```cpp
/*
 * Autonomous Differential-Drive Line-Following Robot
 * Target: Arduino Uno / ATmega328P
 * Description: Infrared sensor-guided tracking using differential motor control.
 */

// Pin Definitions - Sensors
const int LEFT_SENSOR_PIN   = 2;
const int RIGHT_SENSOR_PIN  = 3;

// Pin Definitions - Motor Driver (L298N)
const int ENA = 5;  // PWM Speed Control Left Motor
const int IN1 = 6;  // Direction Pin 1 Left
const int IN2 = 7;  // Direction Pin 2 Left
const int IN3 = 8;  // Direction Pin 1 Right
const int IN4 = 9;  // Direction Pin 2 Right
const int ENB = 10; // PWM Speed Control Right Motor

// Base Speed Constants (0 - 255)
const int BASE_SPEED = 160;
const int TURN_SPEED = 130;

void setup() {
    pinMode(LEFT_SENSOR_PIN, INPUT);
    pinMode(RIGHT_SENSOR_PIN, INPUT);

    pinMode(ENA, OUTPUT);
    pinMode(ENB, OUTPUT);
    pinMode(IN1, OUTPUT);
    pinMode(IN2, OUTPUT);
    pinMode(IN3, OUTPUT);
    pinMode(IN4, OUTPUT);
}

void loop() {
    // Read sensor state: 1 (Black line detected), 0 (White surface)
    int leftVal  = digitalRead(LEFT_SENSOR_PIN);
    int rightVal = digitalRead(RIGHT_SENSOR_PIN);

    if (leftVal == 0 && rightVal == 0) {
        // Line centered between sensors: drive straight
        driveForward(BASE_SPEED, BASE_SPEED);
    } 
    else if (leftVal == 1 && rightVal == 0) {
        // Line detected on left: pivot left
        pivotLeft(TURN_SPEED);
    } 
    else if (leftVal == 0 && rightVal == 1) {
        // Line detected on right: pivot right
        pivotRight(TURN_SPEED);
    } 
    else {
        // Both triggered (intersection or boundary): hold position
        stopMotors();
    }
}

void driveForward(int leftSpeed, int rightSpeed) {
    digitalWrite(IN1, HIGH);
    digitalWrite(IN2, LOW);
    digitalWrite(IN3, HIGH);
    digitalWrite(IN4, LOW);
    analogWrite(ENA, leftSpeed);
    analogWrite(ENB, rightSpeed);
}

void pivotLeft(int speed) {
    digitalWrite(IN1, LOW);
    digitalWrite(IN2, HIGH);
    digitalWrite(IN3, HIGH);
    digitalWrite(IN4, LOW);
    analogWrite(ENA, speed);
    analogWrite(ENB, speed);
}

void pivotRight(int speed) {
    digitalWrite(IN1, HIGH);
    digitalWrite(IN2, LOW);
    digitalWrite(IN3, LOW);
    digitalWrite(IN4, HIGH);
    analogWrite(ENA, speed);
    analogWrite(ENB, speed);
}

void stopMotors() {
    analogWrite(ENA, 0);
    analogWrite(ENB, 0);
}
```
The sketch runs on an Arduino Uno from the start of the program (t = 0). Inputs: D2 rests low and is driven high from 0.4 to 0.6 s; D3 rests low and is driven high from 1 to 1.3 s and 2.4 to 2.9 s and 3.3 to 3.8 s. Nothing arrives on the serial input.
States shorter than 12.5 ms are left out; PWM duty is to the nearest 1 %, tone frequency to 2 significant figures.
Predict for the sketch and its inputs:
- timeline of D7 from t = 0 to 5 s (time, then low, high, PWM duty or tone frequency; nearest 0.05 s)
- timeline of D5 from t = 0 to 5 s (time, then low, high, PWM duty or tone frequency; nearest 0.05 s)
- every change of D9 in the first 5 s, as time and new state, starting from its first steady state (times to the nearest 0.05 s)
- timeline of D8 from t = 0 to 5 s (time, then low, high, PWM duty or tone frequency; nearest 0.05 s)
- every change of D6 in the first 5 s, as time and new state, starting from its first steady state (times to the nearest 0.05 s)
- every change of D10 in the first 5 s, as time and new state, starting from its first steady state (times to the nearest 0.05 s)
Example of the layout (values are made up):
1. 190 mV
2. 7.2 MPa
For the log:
1. 0 s low; 0.4 s high; 0.6 s low
2. 0 s PWM 63 %; 0.4 s PWM 51 %; 0.6 s PWM 63 %; 1 s PWM 51 %; 1.3 s PWM 63 %; 2.4 s PWM 51 %; 2.9 s PWM 63 %; 3.3 s PWM 51 %; 3.8 s PWM 63 %
3. 0 s low; 1 s high; 1.3 s low; 2.4 s high; 2.9 s low; 3.3 s high; 3.8 s low
4. 0 s high; 1 s low; 1.3 s high; 2.4 s low; 2.9 s high; 3.3 s low; 3.8 s high
5. 0 s high; 0.4 s low; 0.6 s high
6. 0 s PWM 63 %; 0.4 s PWM 51 %; 0.6 s PWM 63 %; 1 s PWM 51 %; 1.3 s PWM 63 %; 2.4 s PWM 51 %; 2.9 s PWM 63 %; 3.3 s PWM 51 %; 3.8 s PWM 63 %
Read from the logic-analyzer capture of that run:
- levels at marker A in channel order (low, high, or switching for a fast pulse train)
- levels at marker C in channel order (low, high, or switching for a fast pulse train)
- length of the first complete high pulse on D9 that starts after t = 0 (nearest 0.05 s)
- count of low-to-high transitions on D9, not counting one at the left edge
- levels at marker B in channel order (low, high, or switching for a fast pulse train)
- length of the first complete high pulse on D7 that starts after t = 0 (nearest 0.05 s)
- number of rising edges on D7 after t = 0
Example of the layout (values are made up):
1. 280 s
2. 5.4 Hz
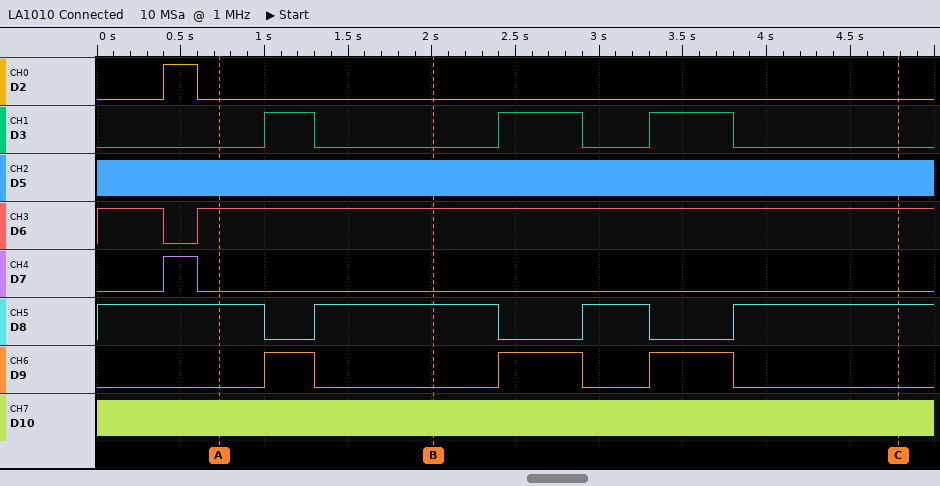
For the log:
1. D2 low, D3 low, D5 switching, D6 high, D7 low, D8 high, D9 low, D10 switching
2. D2 low, D3 low, D5 switching, D6 high, D7 low, D8 high, D9 low, D10 switching
3. 0.30 s
4. 3
5. D2 low, D3 low, D5 switching, D6 high, D7 low, D8 high, D9 low, D10 switching
6. 0.20 s
7. 1
